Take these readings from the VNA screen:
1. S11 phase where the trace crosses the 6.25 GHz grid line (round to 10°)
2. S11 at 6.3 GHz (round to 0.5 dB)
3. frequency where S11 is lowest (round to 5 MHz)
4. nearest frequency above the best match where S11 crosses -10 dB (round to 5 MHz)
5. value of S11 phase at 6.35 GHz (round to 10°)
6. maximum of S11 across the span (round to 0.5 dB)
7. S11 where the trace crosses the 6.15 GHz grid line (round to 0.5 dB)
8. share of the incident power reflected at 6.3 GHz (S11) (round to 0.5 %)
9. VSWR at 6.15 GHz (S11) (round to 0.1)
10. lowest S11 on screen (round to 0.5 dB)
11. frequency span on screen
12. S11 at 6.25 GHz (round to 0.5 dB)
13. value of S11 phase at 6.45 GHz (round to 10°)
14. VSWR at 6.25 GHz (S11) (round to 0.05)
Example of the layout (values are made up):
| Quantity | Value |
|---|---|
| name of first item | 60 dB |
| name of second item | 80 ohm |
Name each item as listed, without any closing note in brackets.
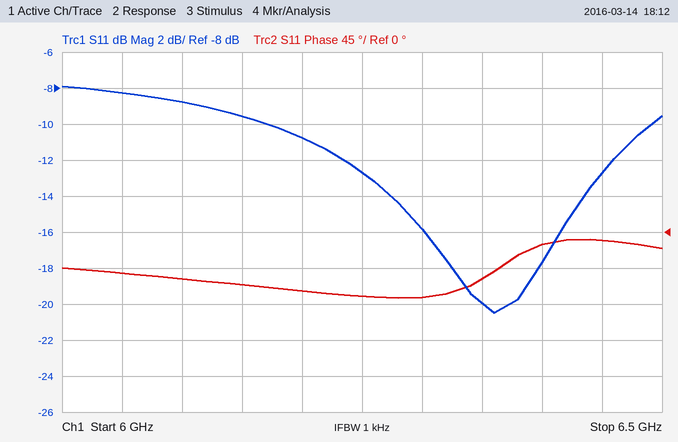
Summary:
| Quantity | Value |
|---|---|
| S11 phase where the trace crosses the 6.25 GHz grid line | -80° |
| S11 at 6.3 GHz | -16.0 dB |
| frequency where S11 is lowest | 6.360 GHz |
| nearest frequency above the best match where S11 crosses -10 dB | 6.490 GHz |
| value of S11 phase at 6.35 GHz | -60° |
| maximum of S11 across the span | -8.0 dB |
| S11 where the trace crosses the 6.15 GHz grid line | -9.5 dB |
| share of the incident power reflected at 6.3 GHz (S11) | 2.5 % |
| VSWR at 6.15 GHz (S11) | 2.0 |
| lowest S11 on screen | -20.5 dB |
| frequency span on screen | 500 MHz |
| S11 at 6.25 GHz | -12.5 dB |
| value of S11 phase at 6.45 GHz | -10° |
| VSWR at 6.25 GHz (S11) | 1.60 |
